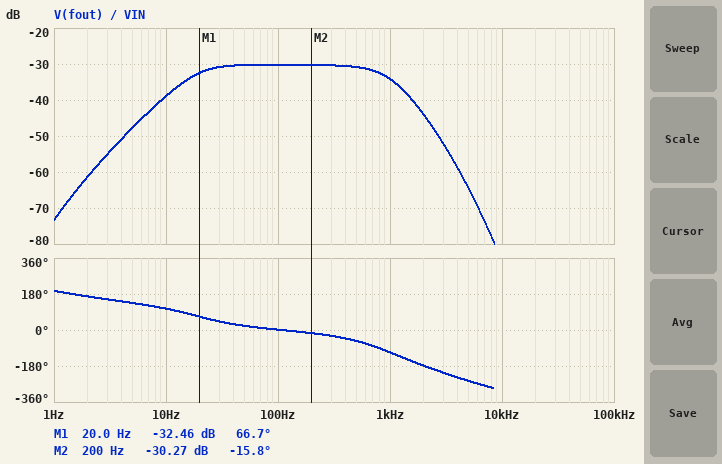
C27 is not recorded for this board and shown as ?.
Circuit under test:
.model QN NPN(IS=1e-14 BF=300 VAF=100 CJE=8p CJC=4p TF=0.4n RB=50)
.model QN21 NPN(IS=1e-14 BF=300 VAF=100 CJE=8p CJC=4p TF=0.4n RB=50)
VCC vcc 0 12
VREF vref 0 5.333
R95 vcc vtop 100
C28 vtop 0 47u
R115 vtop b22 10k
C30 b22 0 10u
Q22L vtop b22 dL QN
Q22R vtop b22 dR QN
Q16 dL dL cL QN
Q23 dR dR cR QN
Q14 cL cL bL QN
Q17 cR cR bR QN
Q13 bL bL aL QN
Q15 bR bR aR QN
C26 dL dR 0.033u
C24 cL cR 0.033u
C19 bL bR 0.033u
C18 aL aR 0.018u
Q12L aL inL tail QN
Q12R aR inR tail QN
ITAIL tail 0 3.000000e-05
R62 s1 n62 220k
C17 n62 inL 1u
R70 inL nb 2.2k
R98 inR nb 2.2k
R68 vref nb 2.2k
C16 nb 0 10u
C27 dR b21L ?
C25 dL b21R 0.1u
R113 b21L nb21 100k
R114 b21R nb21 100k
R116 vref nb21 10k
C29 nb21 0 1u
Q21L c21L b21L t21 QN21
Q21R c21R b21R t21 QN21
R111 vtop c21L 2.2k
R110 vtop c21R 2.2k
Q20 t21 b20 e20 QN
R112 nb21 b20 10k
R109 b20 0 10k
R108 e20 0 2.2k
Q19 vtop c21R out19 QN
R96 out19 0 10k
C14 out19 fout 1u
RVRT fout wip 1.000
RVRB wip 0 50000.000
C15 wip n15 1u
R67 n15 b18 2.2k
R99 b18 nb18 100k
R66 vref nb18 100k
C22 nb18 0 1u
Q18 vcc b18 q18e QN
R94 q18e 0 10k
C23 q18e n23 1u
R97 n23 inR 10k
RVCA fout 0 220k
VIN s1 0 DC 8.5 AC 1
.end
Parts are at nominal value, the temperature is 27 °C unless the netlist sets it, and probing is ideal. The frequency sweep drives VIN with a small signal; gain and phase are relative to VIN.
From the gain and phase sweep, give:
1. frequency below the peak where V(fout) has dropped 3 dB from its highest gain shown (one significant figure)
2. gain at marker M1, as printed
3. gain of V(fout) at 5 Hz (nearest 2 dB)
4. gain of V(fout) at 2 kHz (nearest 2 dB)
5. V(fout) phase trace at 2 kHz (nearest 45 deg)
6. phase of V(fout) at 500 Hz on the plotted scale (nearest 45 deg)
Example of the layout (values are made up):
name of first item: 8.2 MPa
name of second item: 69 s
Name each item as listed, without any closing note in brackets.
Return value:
frequency below the peak where V(fout) has dropped 3 dB from its highest gain shown: 20 Hz
gain at marker M1, as printed: -32.46 dB
gain of V(fout) at 5 Hz: -48 dB
gain of V(fout) at 2 kHz: -44 dB
V(fout) phase trace at 2 kHz: -180 deg
phase of V(fout) at 500 Hz on the plotted scale: -45 deg
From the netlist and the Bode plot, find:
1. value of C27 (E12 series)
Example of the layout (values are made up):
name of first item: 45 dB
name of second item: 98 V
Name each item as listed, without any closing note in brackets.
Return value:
value of C27: 47 nF
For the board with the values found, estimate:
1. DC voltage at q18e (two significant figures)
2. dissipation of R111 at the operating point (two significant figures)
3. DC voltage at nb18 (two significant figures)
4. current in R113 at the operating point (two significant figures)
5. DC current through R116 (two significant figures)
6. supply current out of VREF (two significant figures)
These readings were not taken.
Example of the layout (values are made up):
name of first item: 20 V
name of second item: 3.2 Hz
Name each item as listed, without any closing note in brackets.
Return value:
DC voltage at q18e: 4.4 V
dissipation of R111 at the operating point: 140 µW
DC voltage at nb18: 5.2 V
current in R113 at the operating point: 780 nA
DC current through R116: 180 µA
supply current out of VREF: 180 µA
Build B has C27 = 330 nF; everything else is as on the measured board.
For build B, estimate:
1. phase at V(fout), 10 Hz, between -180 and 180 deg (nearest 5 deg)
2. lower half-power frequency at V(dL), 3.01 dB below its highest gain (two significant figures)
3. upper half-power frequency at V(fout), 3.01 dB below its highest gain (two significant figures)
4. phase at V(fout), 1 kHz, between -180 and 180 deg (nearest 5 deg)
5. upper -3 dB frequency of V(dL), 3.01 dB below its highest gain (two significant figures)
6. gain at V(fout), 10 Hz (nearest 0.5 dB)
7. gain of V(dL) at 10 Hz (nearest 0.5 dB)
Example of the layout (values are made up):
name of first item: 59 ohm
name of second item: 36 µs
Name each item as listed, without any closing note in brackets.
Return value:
phase at V(fout), 10 Hz, between -180 and 180 deg: 85 deg
lower half-power frequency at V(dL), 3.01 dB below its highest gain: 1.7 Hz
upper half-power frequency at V(fout), 3.01 dB below its highest gain: 520 Hz
phase at V(fout), 1 kHz, between -180 and 180 deg: -115 deg
upper -3 dB frequency of V(dL), 3.01 dB below its highest gain: 22 Hz
gain at V(fout), 10 Hz: -31.0 dB
gain of V(dL) at 10 Hz: -44.0 dB
